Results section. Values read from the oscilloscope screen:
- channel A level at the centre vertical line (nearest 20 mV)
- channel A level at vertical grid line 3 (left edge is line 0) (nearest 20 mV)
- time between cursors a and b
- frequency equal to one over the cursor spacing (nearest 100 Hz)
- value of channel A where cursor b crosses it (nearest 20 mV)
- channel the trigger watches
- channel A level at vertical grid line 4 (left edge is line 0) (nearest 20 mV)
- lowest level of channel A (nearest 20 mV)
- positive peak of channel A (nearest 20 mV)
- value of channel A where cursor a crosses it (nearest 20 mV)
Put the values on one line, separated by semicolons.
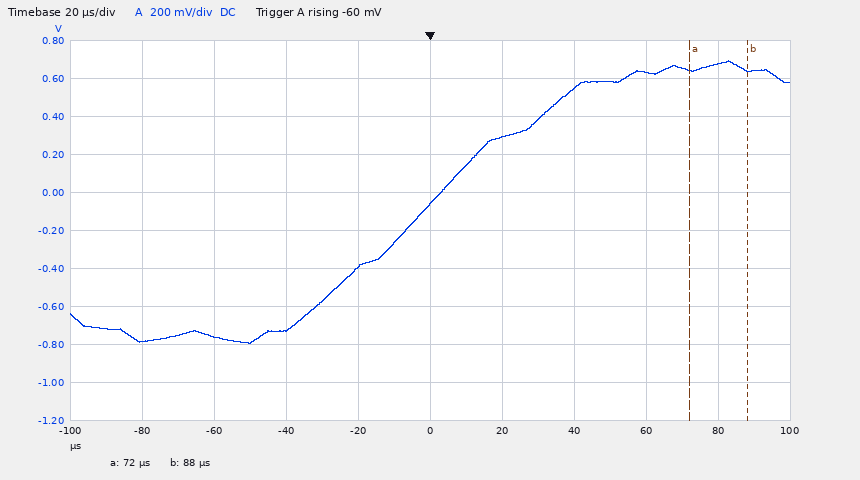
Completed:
-60 mV; -720 mV; 16 µs; 62.5 kHz; 640 mV; channel A; -400 mV; -800 mV; 700 mV; 640 mV
